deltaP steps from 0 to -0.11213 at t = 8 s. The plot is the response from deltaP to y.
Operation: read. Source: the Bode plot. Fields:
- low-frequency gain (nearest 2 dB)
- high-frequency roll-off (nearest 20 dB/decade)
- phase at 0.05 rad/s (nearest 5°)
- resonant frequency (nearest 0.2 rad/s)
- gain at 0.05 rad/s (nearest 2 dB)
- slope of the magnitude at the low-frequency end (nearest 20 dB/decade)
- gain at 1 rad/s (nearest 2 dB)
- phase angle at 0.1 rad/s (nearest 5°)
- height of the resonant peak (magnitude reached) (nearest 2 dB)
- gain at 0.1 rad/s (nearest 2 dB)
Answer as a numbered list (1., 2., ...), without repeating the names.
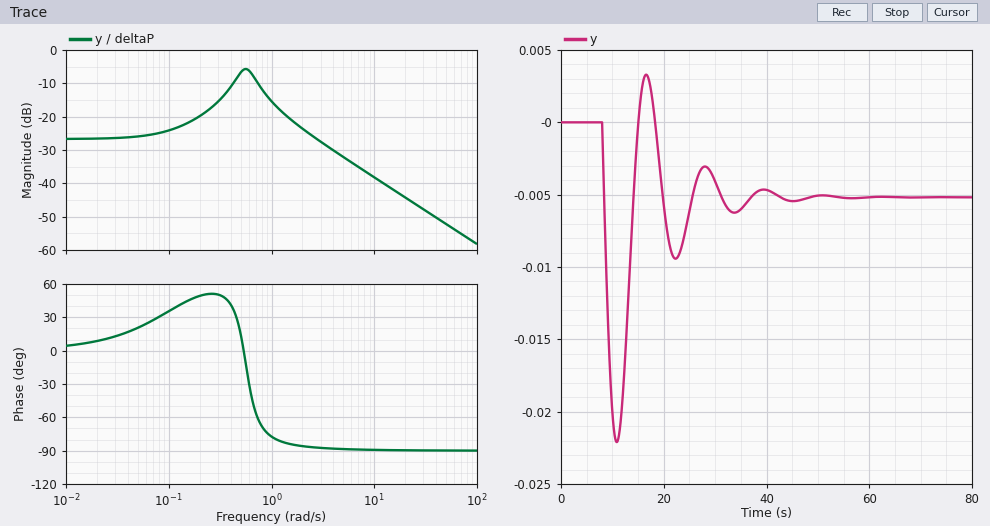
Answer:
1. -26 dB
2. -20 dB/decade
3. 20°
4. 0.6 rad/s
5. -26 dB
6. 0 dB/decade
7. -16 dB
8. 35°
9. -6 dB
10. -24 dB
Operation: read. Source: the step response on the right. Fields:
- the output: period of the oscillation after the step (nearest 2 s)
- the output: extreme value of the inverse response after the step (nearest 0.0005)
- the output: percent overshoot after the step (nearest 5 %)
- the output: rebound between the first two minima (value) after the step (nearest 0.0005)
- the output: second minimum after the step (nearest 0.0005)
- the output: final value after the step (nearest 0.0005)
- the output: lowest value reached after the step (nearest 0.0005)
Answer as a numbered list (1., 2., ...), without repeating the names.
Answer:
1. 12 s
2. 0.0035
3. 325 %
4. 0.0035
5. -0.0095
6. -0.0050
7. -0.0220
